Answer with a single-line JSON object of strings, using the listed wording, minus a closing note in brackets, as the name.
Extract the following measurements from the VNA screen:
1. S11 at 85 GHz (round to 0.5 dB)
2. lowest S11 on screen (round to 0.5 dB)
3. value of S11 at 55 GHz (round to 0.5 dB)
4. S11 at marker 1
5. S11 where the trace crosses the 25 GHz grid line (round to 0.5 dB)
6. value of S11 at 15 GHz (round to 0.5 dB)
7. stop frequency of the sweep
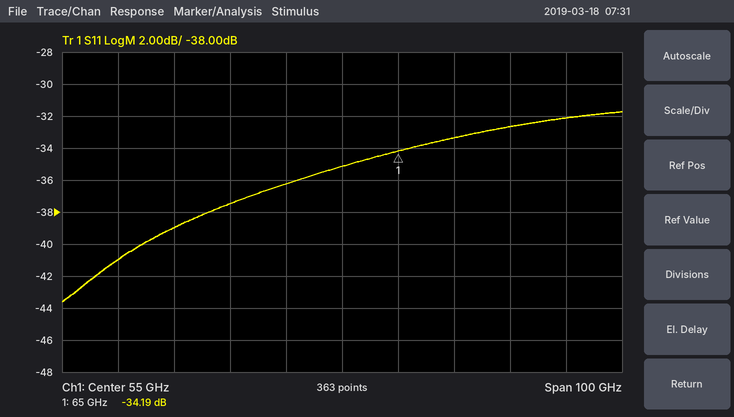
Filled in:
{"S11 at 85 GHz": "-32.5 dB", "lowest S11 on screen": "-43.5 dB", "value of S11 at 55 GHz": "-35.0 dB", "S11 at marker 1": "-34.19 dB", "S11 where the trace crosses the 25 GHz grid line": "-39.0 dB", "value of S11 at 15 GHz": "-41.0 dB", "stop frequency of the sweep": "105 GHz"}
